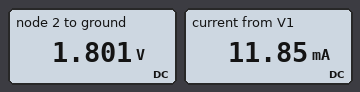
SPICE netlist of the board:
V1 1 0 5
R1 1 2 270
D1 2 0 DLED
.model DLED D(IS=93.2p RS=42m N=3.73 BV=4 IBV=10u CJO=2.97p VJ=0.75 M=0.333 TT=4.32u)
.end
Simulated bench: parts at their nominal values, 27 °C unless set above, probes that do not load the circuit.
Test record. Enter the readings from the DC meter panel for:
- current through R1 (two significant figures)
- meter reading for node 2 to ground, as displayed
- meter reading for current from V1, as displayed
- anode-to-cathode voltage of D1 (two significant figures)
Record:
12 mA
1.801 V
11.85 mA
1.8 V
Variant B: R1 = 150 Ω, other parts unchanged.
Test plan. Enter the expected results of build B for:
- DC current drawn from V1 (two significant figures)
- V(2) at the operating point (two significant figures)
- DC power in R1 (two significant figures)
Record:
21 mA
1.9 V
66 mW
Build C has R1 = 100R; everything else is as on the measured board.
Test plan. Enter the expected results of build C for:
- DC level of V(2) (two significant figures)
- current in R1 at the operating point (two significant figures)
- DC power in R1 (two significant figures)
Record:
1.9 V
31 mA
96 mW
